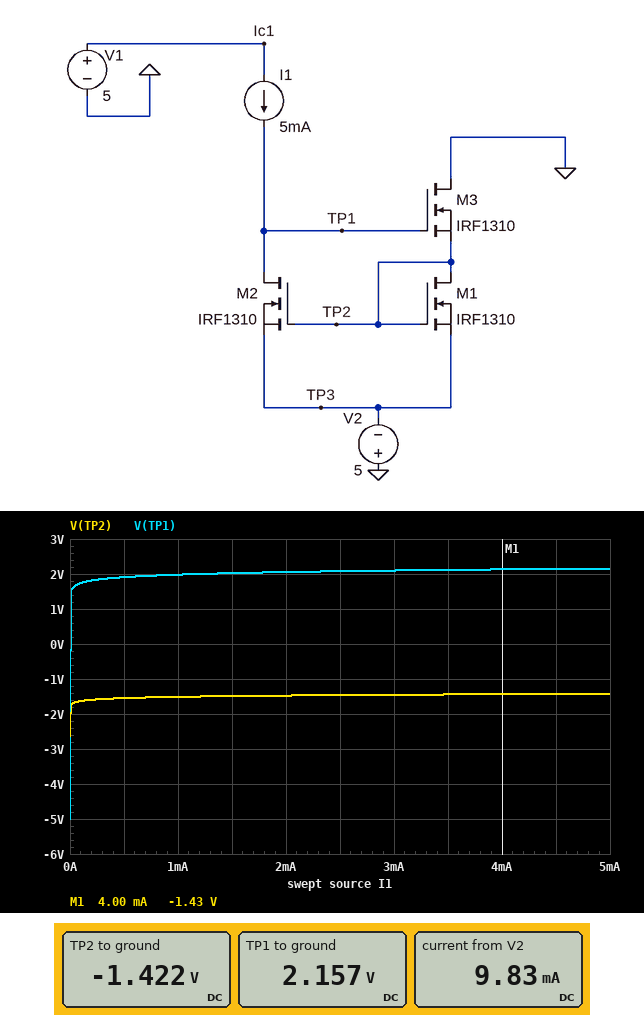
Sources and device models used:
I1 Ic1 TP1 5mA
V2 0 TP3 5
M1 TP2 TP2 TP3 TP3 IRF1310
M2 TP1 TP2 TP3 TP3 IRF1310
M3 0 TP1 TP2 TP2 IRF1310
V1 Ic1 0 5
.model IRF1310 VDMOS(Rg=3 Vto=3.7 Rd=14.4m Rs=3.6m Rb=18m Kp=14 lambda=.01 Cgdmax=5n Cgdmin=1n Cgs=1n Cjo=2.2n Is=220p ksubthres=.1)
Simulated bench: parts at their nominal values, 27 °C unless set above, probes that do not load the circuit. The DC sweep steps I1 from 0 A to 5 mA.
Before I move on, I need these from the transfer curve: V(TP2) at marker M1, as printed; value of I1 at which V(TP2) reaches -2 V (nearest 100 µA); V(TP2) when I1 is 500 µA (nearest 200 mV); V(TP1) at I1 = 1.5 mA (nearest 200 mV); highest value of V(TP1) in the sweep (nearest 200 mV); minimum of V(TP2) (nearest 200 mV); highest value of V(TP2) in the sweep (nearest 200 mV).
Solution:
-1.43 V
0 A
-1.6 V
2.0 V
2.2 V
-2.6 V
-1.4 V
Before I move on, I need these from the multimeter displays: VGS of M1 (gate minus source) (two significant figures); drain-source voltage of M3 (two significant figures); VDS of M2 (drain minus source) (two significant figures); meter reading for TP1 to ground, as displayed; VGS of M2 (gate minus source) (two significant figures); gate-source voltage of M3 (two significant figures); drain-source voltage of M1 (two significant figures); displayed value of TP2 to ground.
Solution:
3.6 V
1.4 V
7.2 V
2.157 V
3.6 V
3.6 V
3.6 V
-1.422 V
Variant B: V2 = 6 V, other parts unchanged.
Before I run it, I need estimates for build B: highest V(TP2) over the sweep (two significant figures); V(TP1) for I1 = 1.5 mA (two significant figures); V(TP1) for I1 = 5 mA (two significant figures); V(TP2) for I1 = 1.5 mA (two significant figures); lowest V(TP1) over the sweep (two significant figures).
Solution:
-2.4 V
1.0 V
1.2 V
-2.5 V
-6.0 V
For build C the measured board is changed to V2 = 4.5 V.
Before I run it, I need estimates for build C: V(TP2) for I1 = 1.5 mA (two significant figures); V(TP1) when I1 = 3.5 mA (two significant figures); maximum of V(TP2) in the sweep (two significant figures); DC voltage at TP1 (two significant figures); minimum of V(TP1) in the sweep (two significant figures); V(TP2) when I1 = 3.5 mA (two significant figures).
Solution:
-990 mV
2.6 V
-920 mV
2.7 V
-4.5 V
-940 mV
